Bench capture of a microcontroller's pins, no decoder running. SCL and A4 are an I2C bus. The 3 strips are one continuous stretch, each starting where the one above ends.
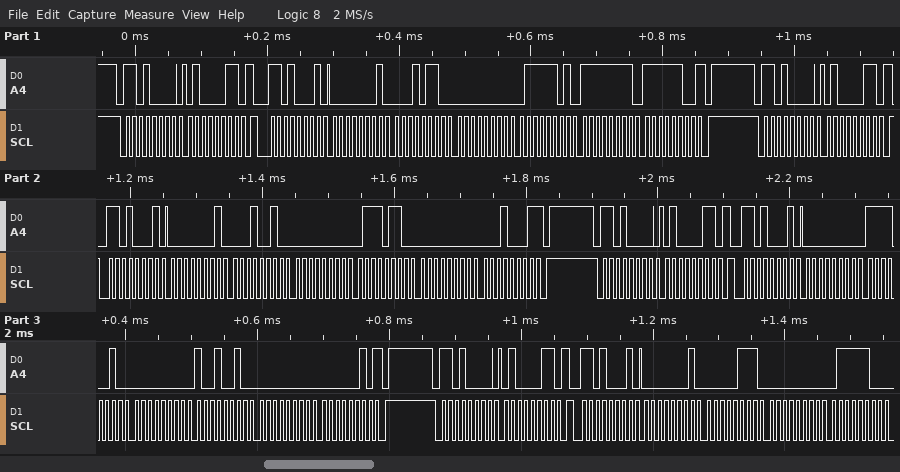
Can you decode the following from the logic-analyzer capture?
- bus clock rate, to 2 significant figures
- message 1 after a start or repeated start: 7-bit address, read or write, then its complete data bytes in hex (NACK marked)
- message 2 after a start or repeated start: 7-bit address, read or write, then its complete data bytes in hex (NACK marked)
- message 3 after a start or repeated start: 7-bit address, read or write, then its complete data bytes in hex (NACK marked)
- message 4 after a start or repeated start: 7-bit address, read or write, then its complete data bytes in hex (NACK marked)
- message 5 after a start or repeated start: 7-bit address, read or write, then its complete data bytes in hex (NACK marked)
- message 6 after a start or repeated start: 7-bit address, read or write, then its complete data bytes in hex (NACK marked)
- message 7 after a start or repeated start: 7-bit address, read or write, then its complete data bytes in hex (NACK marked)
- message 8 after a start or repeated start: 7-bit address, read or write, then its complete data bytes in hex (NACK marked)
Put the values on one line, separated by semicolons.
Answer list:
100 kHz; 0x68 write: 43; 0x68 read: 01 16 00 7D FF FC NACK; 0x68 write: 43; 0x68 read: 01 12 00 76 00 11 NACK; 0x68 write: 43; 0x68 read: 00 F2 00 92 00 02 NACK; 0x68 write: 43; 0x68 read: 01 07 00 7C
